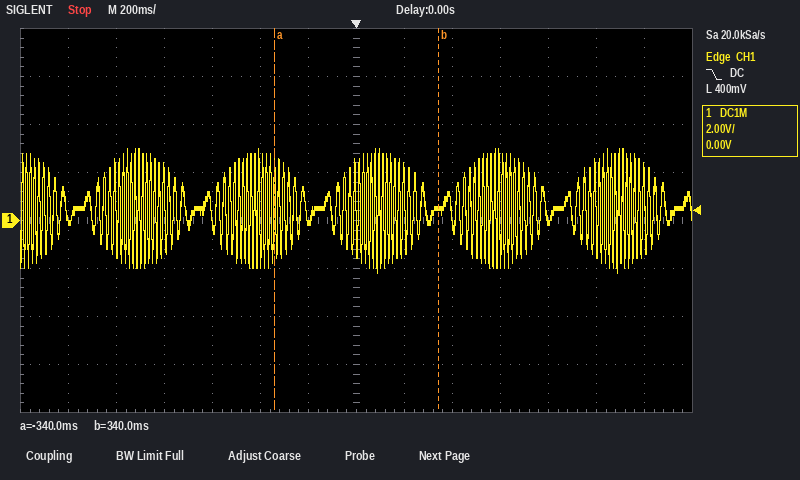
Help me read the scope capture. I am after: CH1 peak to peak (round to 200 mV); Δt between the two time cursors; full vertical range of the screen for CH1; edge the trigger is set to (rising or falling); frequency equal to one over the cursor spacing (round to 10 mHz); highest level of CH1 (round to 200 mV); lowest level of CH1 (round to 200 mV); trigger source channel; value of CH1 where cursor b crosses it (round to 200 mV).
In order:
5.2 V
680 ms
16 V
falling
1.47 Hz
3.0 V
-2.2 V
CH1
400 mV
